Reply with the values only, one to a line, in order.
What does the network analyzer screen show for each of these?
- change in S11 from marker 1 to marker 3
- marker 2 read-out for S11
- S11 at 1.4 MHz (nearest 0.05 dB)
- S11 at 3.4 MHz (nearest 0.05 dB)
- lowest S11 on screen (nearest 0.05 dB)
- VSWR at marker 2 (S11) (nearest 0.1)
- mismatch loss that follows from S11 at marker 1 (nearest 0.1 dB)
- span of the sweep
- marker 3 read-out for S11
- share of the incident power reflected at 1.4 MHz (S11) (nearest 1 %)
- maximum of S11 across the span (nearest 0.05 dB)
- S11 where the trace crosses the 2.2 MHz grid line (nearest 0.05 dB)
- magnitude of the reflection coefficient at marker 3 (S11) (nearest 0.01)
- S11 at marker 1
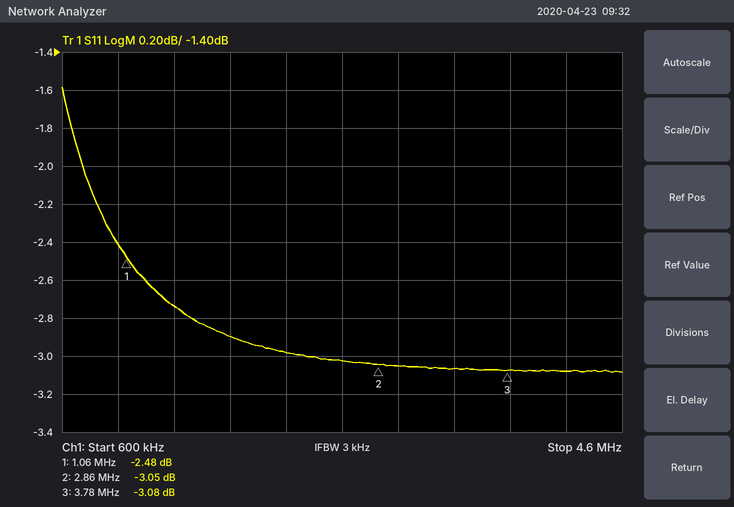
-0.60 dB
-3.05 dB
-2.75 dB
-3.05 dB
-3.10 dB
5.8
3.6 dB
4 MHz
-3.08 dB
53 %
-1.60 dB
-3.00 dB
0.70
-2.48 dB
